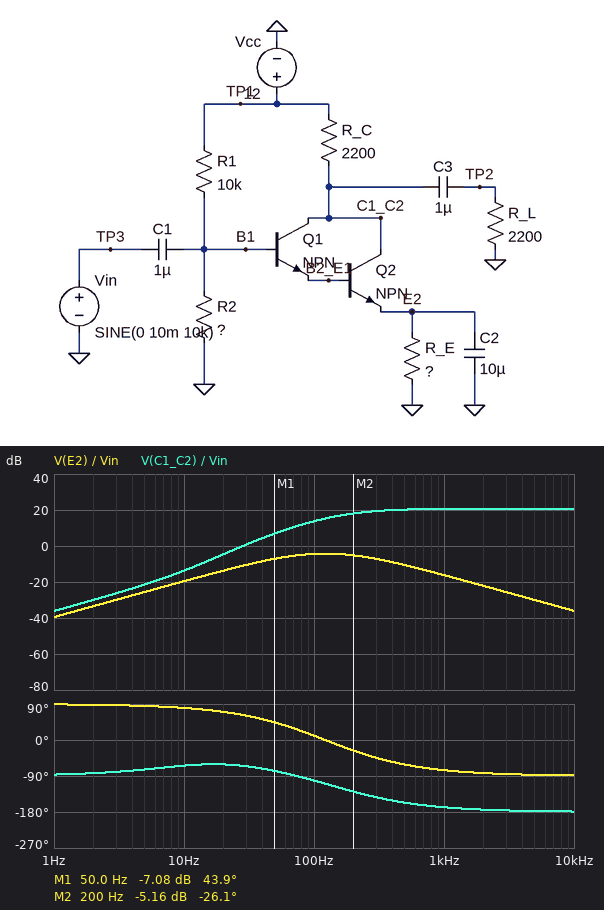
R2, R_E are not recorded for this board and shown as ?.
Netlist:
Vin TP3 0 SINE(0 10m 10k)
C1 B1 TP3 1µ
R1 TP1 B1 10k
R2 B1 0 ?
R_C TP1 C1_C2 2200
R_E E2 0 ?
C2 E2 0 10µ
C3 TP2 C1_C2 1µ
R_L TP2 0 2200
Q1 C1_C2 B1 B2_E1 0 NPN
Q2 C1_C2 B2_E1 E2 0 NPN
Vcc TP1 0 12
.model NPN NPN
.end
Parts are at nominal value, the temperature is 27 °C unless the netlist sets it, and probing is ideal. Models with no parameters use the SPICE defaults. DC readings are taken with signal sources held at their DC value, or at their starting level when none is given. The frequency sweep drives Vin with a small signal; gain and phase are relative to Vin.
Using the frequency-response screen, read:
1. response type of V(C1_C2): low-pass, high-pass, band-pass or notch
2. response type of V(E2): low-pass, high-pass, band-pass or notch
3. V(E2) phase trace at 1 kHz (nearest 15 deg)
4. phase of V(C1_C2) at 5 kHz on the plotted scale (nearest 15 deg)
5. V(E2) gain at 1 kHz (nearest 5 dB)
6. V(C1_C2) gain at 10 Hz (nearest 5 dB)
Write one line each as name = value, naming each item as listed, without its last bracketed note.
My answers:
response type of V(C1_C2): low-pass, high-pass, band-pass or notch = high-pass
response type of V(E2): low-pass, high-pass, band-pass or notch = band-pass
V(E2) phase trace at 1 kHz = -75 deg
phase of V(C1_C2) at 5 kHz on the plotted scale = -180 deg
V(E2) gain at 1 kHz = -15 dB
V(C1_C2) gain at 10 Hz = -15 dB
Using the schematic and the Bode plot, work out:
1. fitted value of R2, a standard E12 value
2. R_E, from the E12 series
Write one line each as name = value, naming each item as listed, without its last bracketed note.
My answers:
fitted value of R2, a standard E12 value = 2.2 kΩ
R_E, from the E12 series = 1.5 kΩ
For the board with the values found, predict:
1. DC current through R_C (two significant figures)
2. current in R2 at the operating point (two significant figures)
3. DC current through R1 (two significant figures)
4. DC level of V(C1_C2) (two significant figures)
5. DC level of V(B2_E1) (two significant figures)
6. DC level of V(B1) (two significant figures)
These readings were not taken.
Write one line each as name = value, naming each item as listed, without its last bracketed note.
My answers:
DC current through R_C = 510 µA
current in R2 at the operating point = 980 µA
DC current through R1 = 980 µA
DC level of V(C1_C2) = 11 V
DC level of V(B2_E1) = 1.5 V
DC level of V(B1) = 2.2 V
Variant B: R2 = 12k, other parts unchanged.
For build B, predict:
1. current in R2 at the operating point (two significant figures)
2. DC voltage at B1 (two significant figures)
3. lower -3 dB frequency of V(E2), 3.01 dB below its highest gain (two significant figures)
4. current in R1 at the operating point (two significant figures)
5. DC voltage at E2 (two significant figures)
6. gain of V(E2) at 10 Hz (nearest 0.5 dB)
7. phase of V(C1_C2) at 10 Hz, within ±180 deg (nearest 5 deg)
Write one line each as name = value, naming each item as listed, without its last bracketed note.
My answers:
current in R2 at the operating point = 510 µA
DC voltage at B1 = 6.1 V
lower -3 dB frequency of V(E2), 3.01 dB below its highest gain = 20 Hz
current in R1 at the operating point = 590 µA
DC voltage at E2 = 4.6 V
gain of V(E2) at 10 Hz = -27.5 dB
phase of V(C1_C2) at 10 Hz, within ±180 deg = 55 deg
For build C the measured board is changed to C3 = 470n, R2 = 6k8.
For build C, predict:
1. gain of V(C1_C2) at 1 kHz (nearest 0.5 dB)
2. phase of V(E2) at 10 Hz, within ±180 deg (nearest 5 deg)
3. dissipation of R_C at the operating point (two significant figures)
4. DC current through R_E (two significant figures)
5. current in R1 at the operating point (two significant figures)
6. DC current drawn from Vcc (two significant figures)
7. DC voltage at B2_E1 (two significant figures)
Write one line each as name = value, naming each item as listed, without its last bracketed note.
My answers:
gain of V(C1_C2) at 1 kHz = 32.0 dB
phase of V(E2) at 10 Hz, within ±180 deg = 75 deg
dissipation of R_C at the operating point = 11 mW
DC current through R_E = 2.3 mA
current in R1 at the operating point = 710 µA
DC current drawn from Vcc = 3.0 mA
DC voltage at B2_E1 = 4.2 V
